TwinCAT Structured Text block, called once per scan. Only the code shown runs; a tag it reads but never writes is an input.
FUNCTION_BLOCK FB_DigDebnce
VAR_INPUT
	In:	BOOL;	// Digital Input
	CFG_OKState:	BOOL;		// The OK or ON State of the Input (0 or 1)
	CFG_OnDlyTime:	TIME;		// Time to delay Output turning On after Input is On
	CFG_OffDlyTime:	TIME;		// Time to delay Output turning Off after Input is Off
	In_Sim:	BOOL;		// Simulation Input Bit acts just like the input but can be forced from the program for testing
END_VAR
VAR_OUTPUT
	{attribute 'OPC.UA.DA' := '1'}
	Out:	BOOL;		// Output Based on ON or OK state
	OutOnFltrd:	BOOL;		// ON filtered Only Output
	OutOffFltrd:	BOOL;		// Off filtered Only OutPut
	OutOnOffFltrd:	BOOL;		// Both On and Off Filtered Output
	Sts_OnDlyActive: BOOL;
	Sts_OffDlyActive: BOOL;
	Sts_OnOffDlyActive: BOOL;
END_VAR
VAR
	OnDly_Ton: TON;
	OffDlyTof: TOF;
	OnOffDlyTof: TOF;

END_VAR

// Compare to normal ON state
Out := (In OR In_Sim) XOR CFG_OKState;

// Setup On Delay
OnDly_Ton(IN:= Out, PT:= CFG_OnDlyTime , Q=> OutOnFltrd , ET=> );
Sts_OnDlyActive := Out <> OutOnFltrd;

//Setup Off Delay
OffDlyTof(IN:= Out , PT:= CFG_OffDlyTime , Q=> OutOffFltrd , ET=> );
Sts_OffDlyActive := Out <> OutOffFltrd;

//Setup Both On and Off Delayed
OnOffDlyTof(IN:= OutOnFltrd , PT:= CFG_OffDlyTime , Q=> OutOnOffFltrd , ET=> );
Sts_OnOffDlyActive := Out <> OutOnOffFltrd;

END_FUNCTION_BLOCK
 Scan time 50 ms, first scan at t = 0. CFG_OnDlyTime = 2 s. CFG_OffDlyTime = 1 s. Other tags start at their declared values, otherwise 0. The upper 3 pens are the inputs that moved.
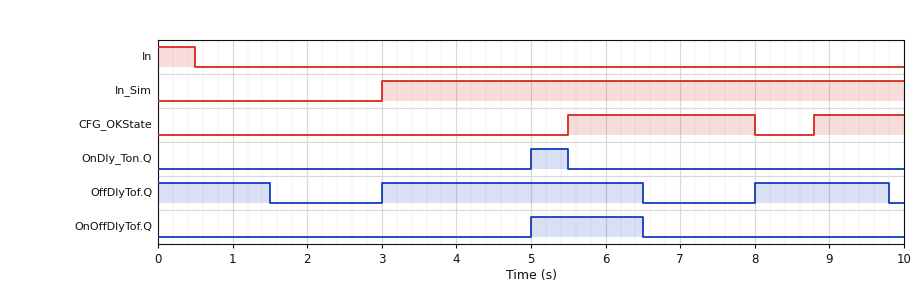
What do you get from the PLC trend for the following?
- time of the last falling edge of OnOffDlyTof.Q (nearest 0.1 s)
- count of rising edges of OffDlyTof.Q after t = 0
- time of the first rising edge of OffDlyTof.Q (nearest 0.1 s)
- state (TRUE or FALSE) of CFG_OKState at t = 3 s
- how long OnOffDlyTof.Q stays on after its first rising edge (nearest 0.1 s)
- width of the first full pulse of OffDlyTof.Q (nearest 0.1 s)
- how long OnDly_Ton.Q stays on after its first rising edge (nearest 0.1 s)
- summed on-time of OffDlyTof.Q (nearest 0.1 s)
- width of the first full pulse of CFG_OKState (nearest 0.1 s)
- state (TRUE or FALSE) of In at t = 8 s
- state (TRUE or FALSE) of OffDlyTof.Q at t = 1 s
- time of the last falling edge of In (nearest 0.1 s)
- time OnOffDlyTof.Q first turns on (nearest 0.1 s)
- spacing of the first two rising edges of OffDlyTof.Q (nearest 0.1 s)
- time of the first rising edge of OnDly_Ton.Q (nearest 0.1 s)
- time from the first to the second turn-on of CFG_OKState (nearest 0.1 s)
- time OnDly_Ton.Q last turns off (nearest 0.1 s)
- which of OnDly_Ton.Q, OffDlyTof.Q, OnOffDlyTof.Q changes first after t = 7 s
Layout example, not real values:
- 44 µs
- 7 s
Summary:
- 6.5 s
- 2
- 3.0 s
- FALSE
- 1.5 s
- 3.5 s
- 0.5 s
- 6.8 s
- 2.5 s
- FALSE
- TRUE
- 0.5 s
- 5.0 s
- 5.0 s
- 5.0 s
- 3.3 s
- 5.5 s
- OffDlyTof.Q
